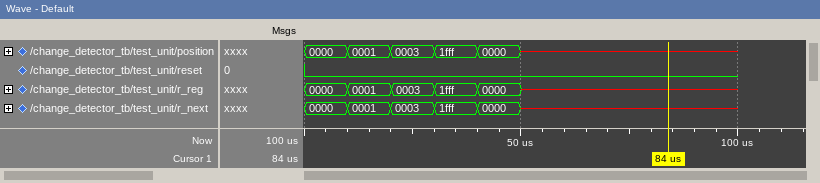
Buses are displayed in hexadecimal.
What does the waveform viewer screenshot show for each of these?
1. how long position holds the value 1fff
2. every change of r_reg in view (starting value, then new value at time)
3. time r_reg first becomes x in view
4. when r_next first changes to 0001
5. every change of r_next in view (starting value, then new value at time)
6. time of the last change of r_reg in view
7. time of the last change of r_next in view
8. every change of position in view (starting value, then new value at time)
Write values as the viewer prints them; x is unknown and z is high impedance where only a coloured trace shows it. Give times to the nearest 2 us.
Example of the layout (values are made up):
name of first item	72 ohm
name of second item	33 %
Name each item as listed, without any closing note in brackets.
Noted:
how long position holds the value 1fff	10 us
every change of r_reg in view	0000, 0001 at 10 us, 0003 at 20 us, 1fff at 30 us, 0000 at 40 us, x at 50 us, x at 60 us
time r_reg first becomes x in view	50 us
when r_next first changes to 0001	10 us
every change of r_next in view	0000, 0001 at 10 us, 0003 at 20 us, 1fff at 30 us, 0000 at 40 us, x at 50 us, x at 60 us
time of the last change of r_reg in view	60 us
time of the last change of r_next in view	60 us
every change of position in view	0000, 0001 at 10 us, 0003 at 20 us, 1fff at 30 us, 0000 at 40 us, x at 50 us, x at 60 us
